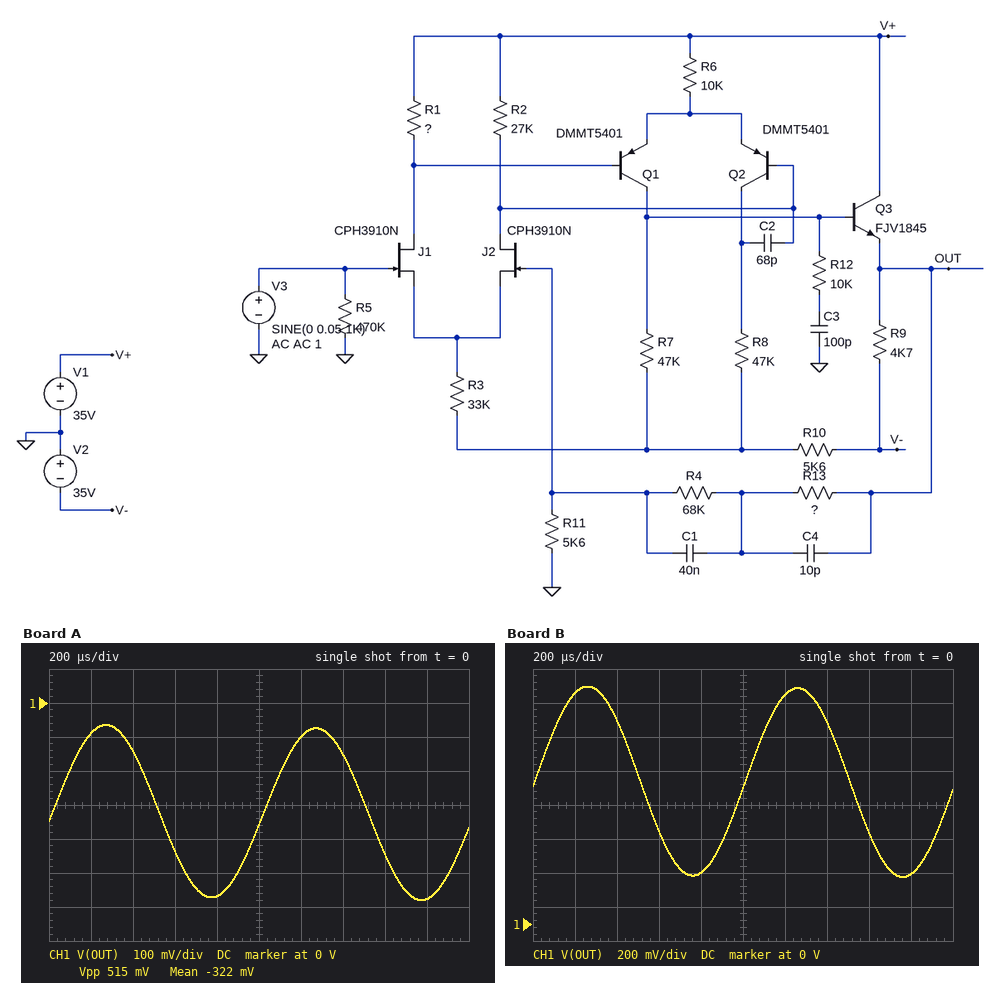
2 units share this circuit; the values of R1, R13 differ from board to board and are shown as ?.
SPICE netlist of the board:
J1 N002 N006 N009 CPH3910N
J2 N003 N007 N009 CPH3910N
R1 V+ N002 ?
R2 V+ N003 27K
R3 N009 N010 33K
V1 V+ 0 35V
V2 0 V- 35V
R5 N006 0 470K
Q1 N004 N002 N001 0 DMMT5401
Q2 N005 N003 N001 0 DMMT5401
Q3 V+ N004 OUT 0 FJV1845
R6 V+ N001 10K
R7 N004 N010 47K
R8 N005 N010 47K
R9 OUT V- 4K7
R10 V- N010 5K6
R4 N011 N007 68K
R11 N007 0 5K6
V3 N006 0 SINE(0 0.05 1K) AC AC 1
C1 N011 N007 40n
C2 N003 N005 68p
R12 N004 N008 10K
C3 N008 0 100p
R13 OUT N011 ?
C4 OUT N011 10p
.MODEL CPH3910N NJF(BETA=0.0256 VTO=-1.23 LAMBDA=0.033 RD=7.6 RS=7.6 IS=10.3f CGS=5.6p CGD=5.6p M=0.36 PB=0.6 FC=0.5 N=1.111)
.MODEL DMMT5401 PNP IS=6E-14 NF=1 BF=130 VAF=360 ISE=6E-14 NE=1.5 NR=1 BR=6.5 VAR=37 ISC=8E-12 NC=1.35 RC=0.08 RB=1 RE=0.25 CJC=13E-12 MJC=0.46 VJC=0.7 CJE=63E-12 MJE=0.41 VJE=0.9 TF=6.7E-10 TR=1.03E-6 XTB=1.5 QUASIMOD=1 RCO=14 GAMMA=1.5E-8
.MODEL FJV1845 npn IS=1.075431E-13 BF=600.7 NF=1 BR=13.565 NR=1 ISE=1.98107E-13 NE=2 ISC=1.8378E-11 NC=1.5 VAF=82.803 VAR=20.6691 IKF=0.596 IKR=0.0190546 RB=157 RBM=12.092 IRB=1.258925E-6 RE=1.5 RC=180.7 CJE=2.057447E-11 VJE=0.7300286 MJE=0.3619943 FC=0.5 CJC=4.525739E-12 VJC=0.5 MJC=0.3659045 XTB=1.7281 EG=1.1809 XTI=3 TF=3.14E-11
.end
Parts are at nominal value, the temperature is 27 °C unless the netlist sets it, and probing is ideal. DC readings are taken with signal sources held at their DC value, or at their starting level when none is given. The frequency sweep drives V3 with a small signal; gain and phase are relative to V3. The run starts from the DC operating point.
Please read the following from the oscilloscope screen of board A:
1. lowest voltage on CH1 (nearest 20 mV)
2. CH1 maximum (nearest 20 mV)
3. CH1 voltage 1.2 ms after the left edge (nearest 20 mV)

-580 mV
-60 mV
-100 mV
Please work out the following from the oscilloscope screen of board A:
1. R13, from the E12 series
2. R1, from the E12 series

22 kΩ
18 kΩ
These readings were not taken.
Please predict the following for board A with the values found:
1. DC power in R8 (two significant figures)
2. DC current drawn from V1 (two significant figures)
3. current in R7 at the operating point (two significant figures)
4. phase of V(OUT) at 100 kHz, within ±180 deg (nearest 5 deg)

2.9 mW
9.0 mA
560 µA
-5 deg
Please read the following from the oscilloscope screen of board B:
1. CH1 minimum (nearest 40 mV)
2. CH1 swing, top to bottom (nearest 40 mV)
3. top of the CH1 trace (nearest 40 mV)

280 mV
1.12 V
1.40 V
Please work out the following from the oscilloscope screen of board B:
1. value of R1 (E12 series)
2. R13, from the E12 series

56 kΩ
56 kΩ
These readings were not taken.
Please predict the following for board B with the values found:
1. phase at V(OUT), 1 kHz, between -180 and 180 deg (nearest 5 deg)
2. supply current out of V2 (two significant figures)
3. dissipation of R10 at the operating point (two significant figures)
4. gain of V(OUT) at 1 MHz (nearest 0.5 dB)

-5 deg
9.6 mA
23 mW
10.5 dB
